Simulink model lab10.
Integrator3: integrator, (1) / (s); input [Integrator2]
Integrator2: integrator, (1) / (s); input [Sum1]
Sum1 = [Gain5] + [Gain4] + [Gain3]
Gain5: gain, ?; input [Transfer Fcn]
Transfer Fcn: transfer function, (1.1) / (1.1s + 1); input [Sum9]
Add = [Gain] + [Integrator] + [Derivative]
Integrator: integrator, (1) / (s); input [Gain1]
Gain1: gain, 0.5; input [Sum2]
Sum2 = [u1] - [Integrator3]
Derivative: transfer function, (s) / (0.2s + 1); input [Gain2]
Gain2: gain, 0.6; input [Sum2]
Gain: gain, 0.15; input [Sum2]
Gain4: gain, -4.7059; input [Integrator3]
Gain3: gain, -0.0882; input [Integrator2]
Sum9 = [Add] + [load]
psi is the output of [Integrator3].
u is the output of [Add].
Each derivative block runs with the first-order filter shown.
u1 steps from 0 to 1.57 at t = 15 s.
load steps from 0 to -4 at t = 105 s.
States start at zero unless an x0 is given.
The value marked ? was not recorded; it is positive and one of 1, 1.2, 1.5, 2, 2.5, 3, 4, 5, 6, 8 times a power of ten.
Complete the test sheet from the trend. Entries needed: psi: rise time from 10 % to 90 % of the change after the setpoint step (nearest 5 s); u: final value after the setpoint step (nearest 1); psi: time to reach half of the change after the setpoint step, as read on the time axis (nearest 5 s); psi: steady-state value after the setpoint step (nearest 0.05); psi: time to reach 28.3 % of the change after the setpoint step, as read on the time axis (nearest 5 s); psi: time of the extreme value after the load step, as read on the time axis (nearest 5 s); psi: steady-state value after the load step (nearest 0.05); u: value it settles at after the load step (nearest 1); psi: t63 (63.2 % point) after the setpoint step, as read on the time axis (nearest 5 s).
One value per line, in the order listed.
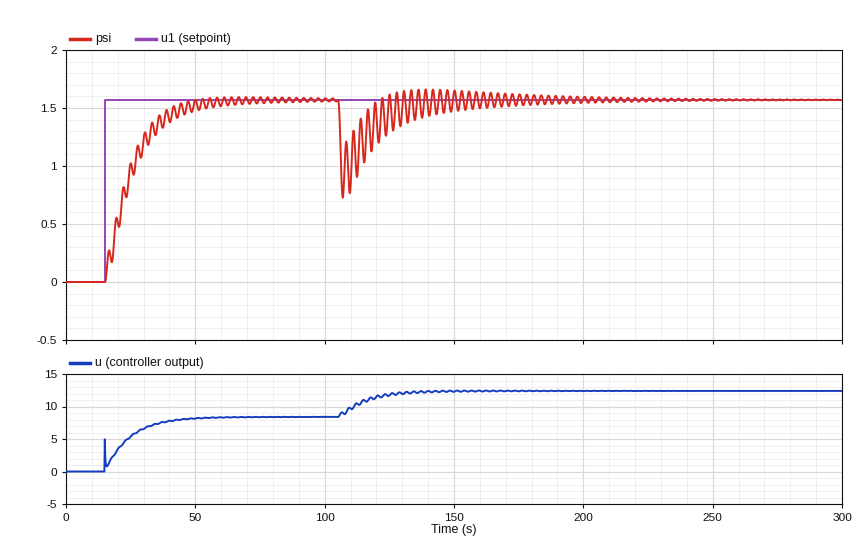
20 s
8
20 s
1.55
20 s
105 s
1.55
12
25 s
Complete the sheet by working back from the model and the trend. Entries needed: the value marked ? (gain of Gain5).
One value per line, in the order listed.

0.8
